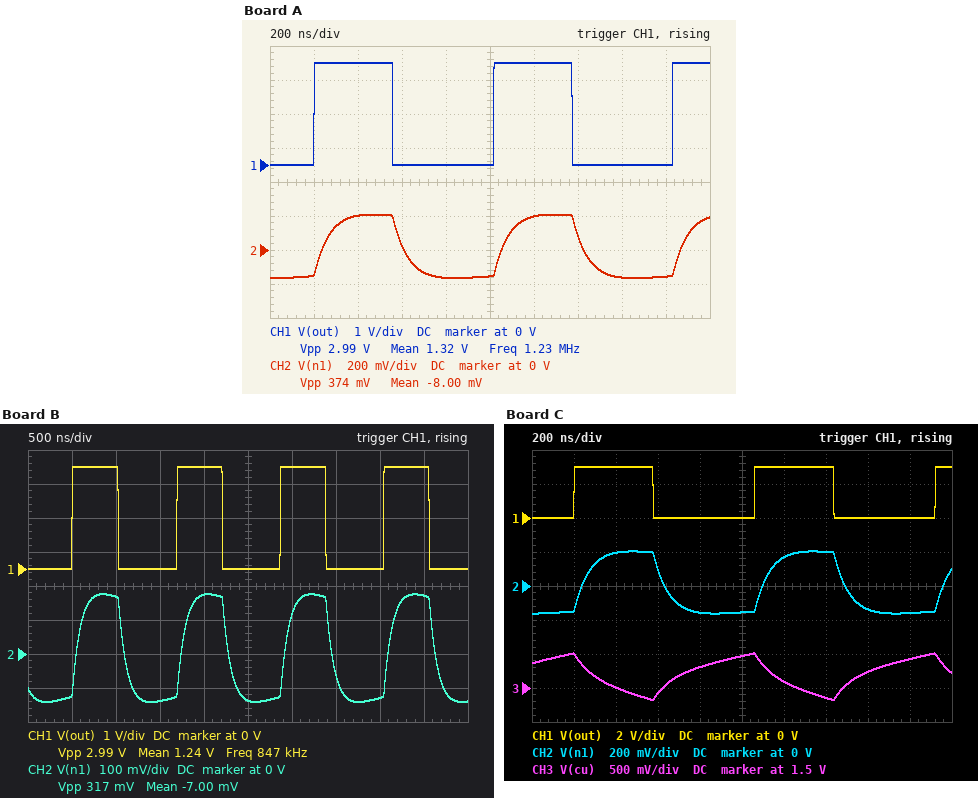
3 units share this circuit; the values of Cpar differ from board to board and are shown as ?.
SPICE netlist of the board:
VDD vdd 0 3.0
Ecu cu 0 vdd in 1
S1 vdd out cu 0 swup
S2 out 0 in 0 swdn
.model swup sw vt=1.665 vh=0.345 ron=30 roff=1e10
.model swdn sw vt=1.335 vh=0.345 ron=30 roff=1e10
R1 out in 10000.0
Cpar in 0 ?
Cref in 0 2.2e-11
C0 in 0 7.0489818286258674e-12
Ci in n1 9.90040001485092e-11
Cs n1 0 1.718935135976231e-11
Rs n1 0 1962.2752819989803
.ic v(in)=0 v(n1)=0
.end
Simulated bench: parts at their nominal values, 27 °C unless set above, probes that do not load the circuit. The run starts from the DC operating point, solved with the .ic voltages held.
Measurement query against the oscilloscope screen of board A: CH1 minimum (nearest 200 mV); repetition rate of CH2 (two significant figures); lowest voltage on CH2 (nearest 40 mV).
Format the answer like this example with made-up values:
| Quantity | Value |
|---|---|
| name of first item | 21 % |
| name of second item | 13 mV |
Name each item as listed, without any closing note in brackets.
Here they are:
| Quantity | Value |
|---|---|
| CH1 minimum | 0 V |
| repetition rate of CH2 | 1.2 MHz |
| lowest voltage on CH2 | -160 mV |
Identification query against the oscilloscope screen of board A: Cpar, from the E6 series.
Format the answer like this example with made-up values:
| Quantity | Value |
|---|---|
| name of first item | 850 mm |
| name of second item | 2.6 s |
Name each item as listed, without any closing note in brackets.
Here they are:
| Quantity | Value |
|---|---|
| Cpar, from the E6 series | 3.3 pF |
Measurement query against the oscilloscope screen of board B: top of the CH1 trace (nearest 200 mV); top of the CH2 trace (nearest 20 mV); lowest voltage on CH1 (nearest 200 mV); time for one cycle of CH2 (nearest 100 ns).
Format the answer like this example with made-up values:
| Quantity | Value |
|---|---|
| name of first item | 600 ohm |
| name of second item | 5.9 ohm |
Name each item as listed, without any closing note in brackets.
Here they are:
| Quantity | Value |
|---|---|
| top of the CH1 trace | 3.0 V |
| top of the CH2 trace | 180 mV |
| lowest voltage on CH1 | 0 V |
| time for one cycle of CH2 | 1.2 µs |
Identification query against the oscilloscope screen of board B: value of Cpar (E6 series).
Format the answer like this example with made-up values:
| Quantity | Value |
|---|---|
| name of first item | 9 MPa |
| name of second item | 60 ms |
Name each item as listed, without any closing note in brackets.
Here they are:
| Quantity | Value |
|---|---|
| value of Cpar | 33 pF |
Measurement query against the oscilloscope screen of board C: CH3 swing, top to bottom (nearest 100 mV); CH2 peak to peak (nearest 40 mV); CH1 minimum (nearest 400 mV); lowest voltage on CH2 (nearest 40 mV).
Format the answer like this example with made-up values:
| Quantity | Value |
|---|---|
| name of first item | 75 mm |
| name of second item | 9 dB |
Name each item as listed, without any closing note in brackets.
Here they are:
| Quantity | Value |
|---|---|
| CH3 swing, top to bottom | 700 mV |
| CH2 peak to peak | 360 mV |
| CH1 minimum | 0 V |
| lowest voltage on CH2 | -160 mV |
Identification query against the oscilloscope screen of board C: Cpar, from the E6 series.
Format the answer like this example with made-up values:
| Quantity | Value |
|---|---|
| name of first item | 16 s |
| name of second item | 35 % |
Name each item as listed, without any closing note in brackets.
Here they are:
| Quantity | Value |
|---|---|
| Cpar, from the E6 series | 6.8 pF |
